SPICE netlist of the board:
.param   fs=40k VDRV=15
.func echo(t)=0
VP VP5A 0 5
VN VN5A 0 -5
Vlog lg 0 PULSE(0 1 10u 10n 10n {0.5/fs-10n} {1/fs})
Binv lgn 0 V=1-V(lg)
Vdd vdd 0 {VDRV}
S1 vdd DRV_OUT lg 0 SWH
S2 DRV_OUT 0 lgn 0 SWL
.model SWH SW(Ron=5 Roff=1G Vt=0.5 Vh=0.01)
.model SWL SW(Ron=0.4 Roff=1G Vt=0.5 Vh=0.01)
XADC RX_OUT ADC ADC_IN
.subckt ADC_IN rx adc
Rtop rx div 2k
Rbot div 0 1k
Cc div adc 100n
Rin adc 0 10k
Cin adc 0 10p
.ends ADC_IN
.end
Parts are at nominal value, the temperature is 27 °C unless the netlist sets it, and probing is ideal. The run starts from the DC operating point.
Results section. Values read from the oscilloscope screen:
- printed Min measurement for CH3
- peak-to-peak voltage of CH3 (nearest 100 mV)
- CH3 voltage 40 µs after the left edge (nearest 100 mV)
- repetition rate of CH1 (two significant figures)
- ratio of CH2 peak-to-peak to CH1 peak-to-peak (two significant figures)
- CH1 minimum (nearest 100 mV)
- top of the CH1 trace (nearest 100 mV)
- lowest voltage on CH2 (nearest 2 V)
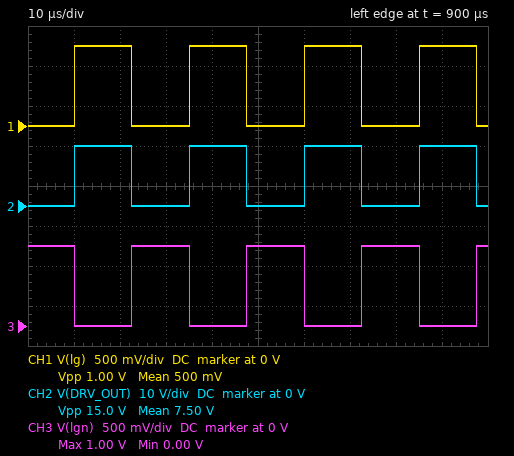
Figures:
0.00 V
1.0 V
0 V
40 kHz
15
0 V
1.0 V
0 V
